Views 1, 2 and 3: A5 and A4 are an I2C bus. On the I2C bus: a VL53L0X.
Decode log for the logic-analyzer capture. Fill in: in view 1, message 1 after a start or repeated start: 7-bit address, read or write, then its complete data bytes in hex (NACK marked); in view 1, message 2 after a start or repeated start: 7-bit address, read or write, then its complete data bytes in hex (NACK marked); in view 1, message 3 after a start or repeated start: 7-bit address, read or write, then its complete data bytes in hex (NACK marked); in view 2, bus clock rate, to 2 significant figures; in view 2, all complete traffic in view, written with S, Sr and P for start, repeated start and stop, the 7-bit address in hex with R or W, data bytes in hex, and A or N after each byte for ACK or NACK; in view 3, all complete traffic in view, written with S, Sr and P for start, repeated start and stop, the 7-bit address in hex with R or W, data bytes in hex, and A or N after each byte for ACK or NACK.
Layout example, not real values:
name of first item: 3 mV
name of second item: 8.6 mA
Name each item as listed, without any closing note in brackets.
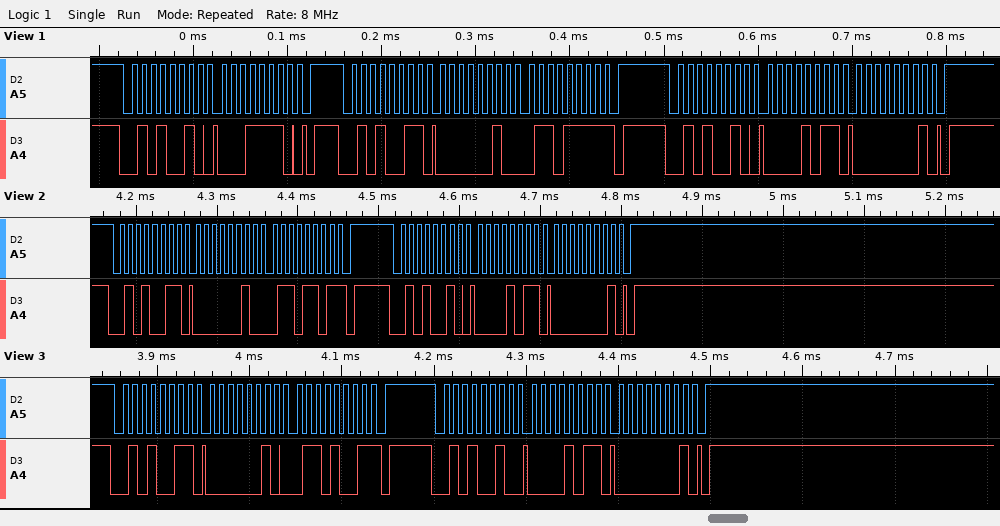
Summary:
in view 1, message 1 after a start or repeated start: 7-bit address, read or write, then its complete data bytes in hex: 0x29 write: 1E
in view 1, message 2 after a start or repeated start: 7-bit address, read or write, then its complete data bytes in hex: 0x29 read: 02 6F NACK
in view 1, message 3 after a start or repeated start: 7-bit address, read or write, then its complete data bytes in hex: 0x29 write: 0B 01
in view 2, bus clock rate, to 2 significant figures: 100 kHz
in view 2, all complete traffic in view, written with S, Sr and P for start, repeated start and stop, the 7-bit address in hex with R or W, data bytes in hex, and A or N after each byte for ACK or NACK: S 29R A 02 A 6D N P S 29W A 0B A 01 A P
in view 3, all complete traffic in view, written with S, Sr and P for start, repeated start and stop, the 7-bit address in hex with R or W, data bytes in hex, and A or N after each byte for ACK or NACK: S 29R A 02 A 69 N P S 29W A 0B A 01 A P
